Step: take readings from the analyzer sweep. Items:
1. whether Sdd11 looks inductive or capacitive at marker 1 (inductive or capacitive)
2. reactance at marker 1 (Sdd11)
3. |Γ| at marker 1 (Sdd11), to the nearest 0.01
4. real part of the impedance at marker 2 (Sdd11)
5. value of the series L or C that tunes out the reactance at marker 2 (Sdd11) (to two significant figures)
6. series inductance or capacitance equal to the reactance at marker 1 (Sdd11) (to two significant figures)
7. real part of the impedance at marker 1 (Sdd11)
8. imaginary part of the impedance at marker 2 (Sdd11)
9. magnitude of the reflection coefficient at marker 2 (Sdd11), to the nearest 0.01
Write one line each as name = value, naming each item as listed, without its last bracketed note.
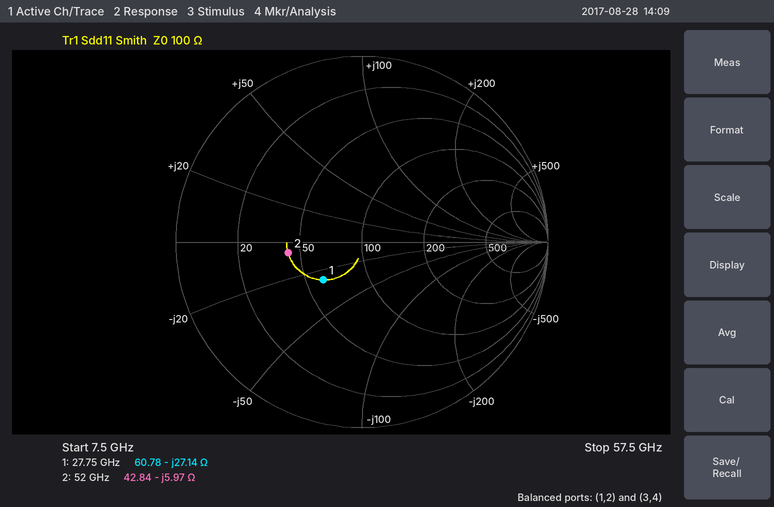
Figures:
whether Sdd11 looks inductive or capacitive at marker 1 = capacitive
reactance at marker 1 = -27.14 Ω
|Γ| at marker 1 (Sdd11), to the nearest 0.01 = 0.29
real part of the impedance at marker 2 = 42.84 Ω
value of the series L or C that tunes out the reactance at marker 2 (Sdd11) = 18 pH
series inductance or capacitance equal to the reactance at marker 1 (Sdd11) = 210 fF
real part of the impedance at marker 1 = 60.78 Ω
imaginary part of the impedance at marker 2 = -5.97 Ω
magnitude of the reflection coefficient at marker 2 (Sdd11), to the nearest 0.01 = 0.40
